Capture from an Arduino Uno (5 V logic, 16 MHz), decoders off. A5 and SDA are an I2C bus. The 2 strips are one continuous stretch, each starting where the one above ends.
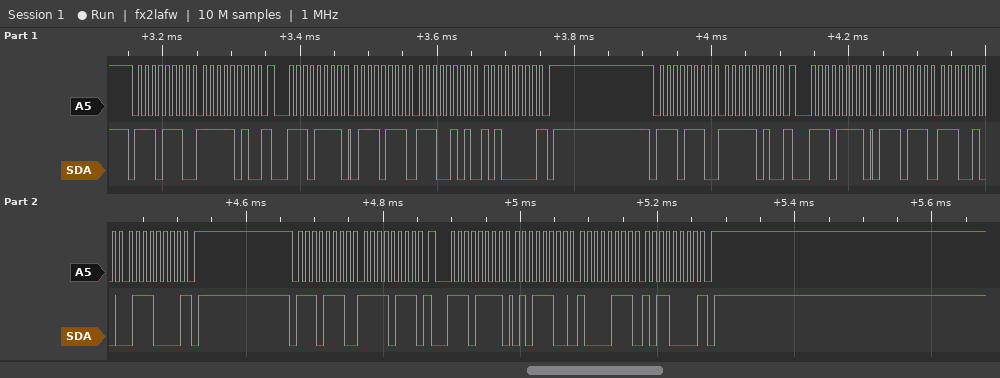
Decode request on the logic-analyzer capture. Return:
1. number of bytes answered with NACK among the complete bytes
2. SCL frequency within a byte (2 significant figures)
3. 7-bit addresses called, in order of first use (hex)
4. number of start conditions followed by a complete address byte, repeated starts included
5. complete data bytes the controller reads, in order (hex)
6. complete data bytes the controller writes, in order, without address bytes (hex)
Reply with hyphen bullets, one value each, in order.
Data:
- 3
- 100 kHz
- 0x77
- 6
- 77 E5 A0 77 E4 70 5C 87 B0
- FA FA F7
